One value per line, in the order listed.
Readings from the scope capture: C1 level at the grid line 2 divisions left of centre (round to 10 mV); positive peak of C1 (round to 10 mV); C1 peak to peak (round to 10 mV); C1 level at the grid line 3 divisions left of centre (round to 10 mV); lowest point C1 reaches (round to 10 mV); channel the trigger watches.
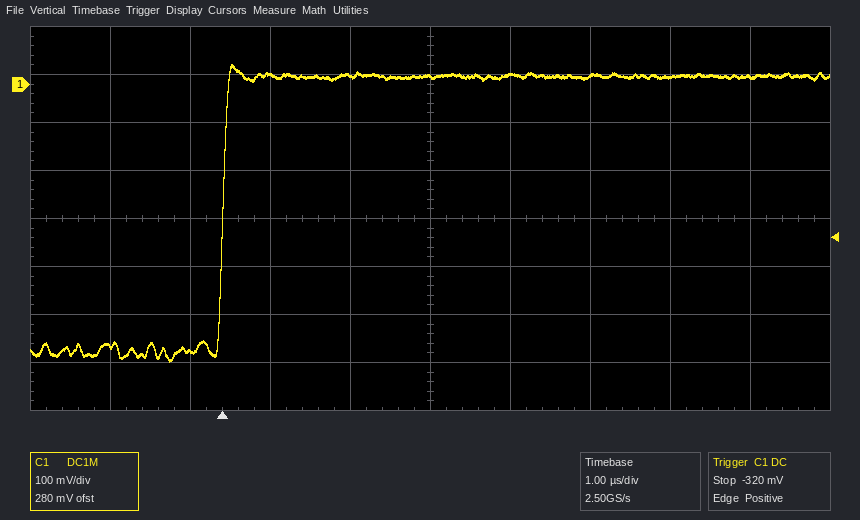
20 mV
40 mV
620 mV
-560 mV
-580 mV
C1
